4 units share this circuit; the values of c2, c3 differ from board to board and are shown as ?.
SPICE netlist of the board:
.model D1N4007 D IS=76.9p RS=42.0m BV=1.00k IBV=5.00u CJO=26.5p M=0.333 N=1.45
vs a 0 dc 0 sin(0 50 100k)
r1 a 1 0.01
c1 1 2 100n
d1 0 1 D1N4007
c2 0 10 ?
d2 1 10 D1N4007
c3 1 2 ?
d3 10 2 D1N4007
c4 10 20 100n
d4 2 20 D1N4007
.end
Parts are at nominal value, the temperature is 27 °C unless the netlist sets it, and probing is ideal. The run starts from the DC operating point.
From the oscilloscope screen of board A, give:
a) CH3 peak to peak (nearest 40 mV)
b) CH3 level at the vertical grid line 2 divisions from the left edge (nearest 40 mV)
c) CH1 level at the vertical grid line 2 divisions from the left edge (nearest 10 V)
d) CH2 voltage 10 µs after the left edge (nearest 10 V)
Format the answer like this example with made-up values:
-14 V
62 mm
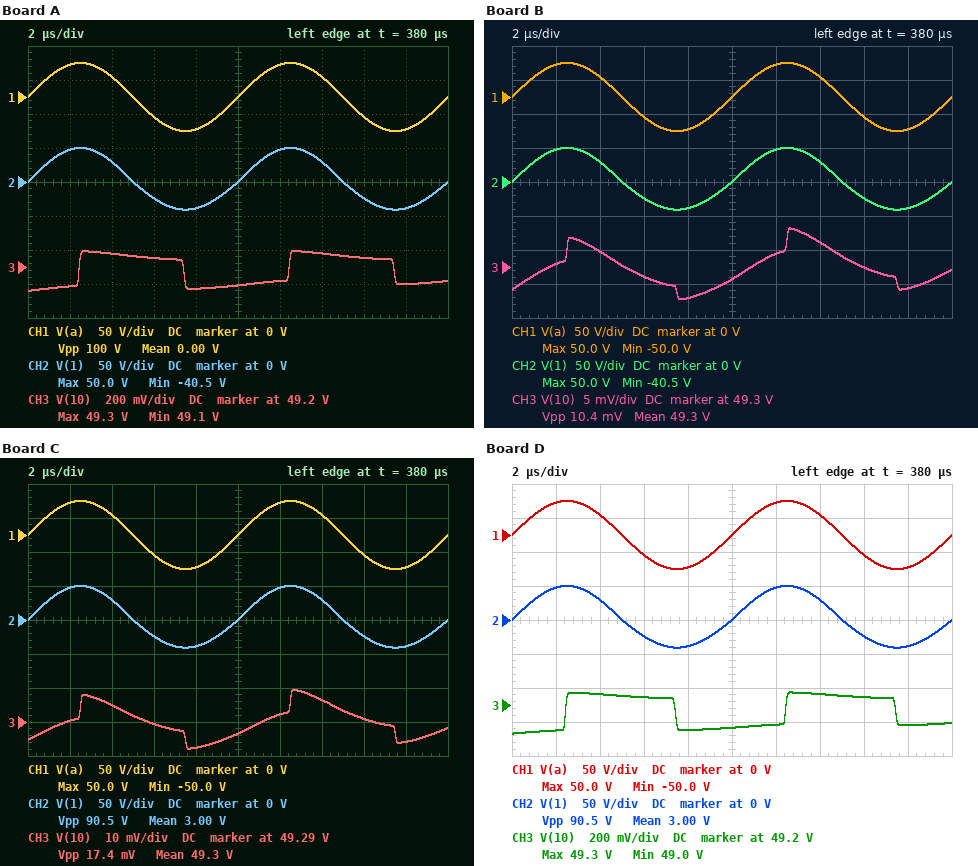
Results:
240 mV
49.28 V
30 V
0 V
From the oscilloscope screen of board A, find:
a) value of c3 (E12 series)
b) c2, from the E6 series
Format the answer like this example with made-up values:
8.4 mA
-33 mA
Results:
47 nF
47 nF
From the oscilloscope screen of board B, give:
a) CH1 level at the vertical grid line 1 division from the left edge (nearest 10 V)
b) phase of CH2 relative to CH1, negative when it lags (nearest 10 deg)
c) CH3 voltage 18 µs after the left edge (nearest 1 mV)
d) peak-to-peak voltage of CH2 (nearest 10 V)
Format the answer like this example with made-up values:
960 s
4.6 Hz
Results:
50 V
0 deg
49.302 V
90 V
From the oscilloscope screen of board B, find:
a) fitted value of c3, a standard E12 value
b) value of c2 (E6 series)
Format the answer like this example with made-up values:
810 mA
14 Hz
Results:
33 nF
330 nF
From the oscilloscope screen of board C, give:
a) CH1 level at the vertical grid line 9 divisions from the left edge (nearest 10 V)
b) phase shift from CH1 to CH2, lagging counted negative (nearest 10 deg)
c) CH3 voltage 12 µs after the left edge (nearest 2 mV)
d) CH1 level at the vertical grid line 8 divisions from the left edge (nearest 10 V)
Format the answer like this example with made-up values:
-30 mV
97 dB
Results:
-50 V
0 deg
49.292 V
-30 V
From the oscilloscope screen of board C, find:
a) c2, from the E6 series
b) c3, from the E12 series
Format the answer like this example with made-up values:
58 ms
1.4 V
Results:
220 nF
150 nF
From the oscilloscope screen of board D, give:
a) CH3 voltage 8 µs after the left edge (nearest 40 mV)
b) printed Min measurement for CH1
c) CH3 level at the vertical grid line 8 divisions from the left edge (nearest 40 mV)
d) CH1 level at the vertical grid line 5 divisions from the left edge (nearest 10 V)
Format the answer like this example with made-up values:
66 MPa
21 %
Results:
49.04 V
-50.0 V
49.24 V
0 V
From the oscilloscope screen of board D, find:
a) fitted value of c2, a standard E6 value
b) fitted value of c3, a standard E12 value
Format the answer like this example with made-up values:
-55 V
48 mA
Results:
68 nF
180 nF
